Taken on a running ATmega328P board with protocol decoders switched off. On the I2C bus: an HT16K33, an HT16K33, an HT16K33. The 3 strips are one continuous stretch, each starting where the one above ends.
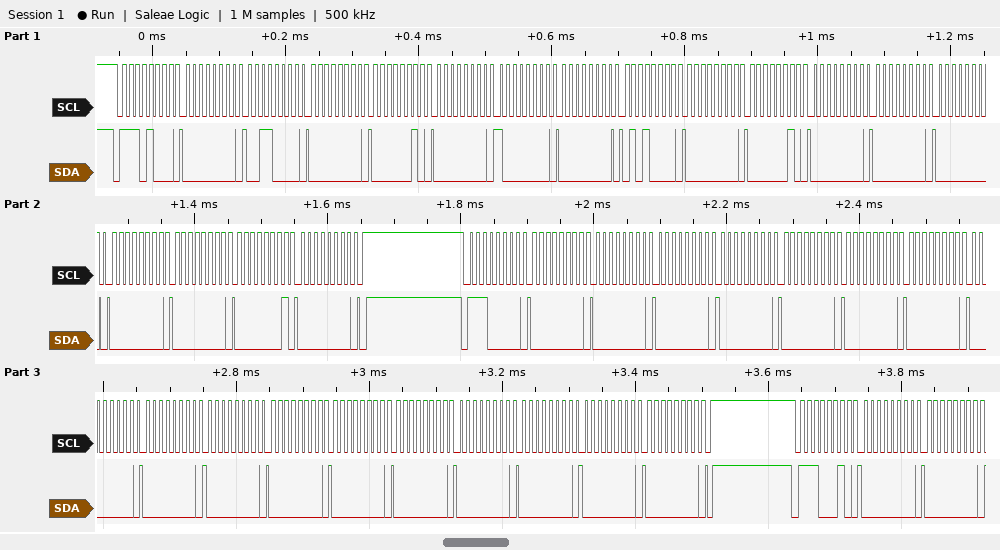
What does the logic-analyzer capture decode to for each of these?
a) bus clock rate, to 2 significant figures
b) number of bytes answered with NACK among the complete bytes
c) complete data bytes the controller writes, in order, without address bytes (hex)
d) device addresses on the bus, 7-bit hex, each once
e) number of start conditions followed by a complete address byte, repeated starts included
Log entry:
100 kHz
0
00 30 00 02 00 80 00 50 00 02 00 00 00 00 00 01 00 00 00 00 00 00 00 00 00 00 00 00 00 00 00 00 00 00 00 00
0x74 0x70 0x71
3
